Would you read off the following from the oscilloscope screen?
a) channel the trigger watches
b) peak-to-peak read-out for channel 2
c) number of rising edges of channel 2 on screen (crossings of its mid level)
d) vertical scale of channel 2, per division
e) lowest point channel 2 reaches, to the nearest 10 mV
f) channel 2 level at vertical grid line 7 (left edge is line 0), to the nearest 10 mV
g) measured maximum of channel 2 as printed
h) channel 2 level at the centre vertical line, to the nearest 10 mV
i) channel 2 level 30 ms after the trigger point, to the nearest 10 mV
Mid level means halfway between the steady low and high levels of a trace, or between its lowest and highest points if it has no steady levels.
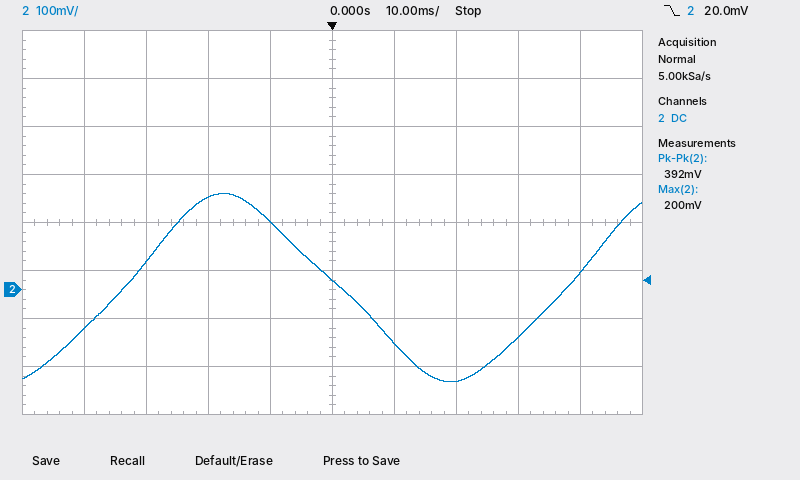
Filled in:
channel 2
392 mV
2
100 mV
-190 mV
-190 mV
200 mV
20 mV
-100 mV
